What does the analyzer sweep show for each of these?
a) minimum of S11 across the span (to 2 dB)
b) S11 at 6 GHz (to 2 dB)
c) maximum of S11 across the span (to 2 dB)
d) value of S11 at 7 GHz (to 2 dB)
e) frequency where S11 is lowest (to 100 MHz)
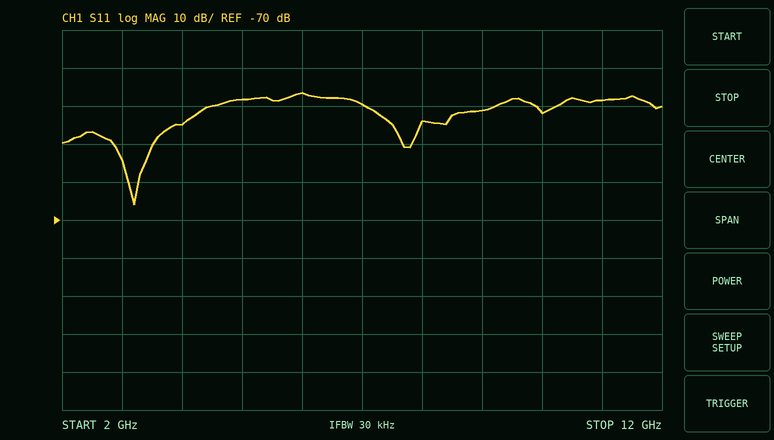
-66 dB
-36 dB
-36 dB
-40 dB
3.2 GHz
